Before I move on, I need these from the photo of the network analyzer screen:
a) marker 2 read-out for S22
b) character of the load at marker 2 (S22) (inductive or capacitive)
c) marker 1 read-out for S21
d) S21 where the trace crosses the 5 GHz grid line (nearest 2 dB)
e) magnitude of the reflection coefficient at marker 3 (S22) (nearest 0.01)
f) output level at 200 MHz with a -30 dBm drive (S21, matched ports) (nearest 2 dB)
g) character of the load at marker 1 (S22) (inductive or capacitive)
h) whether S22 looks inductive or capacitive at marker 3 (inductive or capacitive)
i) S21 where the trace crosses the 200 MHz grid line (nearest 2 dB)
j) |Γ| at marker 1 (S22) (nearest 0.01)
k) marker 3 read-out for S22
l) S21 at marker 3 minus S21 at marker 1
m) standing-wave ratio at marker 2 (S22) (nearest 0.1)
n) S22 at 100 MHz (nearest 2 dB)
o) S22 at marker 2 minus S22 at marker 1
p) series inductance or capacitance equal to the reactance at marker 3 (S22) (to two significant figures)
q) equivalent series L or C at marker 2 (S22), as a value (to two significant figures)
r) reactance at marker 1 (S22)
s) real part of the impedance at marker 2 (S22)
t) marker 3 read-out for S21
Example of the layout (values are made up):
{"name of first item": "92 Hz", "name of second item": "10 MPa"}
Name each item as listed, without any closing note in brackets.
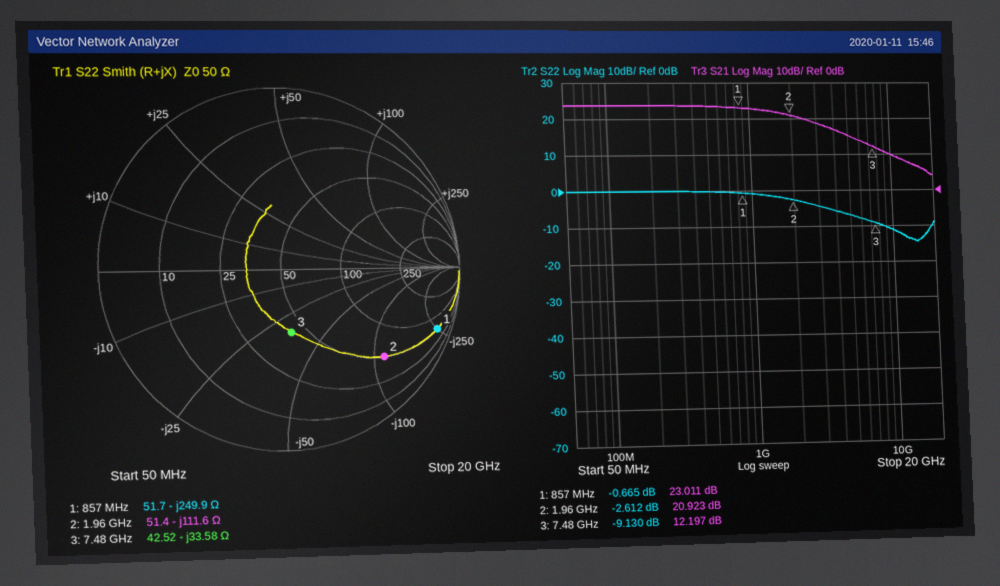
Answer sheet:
{"marker 2 read-out for S22": "-2.612 dB", "character of the load at marker 2 (S22)": "capacitive", "marker 1 read-out for S21": "23.011 dB", "S21 where the trace crosses the 5 GHz grid line": "16 dB", "magnitude of the reflection coefficient at marker 3 (S22)": "0.35", "output level at 200 MHz with a -30 dBm drive (S21, matched ports)": "-6 dBm", "character of the load at marker 1 (S22)": "capacitive", "whether S22 looks inductive or capacitive at marker 3": "capacitive", "S21 where the trace crosses the 200 MHz grid line": "24 dB", "|Γ| at marker 1 (S22)": "0.93", "marker 3 read-out for S22": "-9.130 dB", "S21 at marker 3 minus S21 at marker 1": "-10.814 dB", "standing-wave ratio at marker 2 (S22)": "6.7", "S22 at 100 MHz": "0 dB", "S22 at marker 2 minus S22 at marker 1": "-1.947 dB", "series inductance or capacitance equal to the reactance at marker 3 (S22)": "630 fF", "equivalent series L or C at marker 2 (S22), as a value": "730 fF", "reactance at marker 1": "-249.9 Ω", "real part of the impedance at marker 2": "51.4 Ω", "marker 3 read-out for S21": "12.197 dB"}
